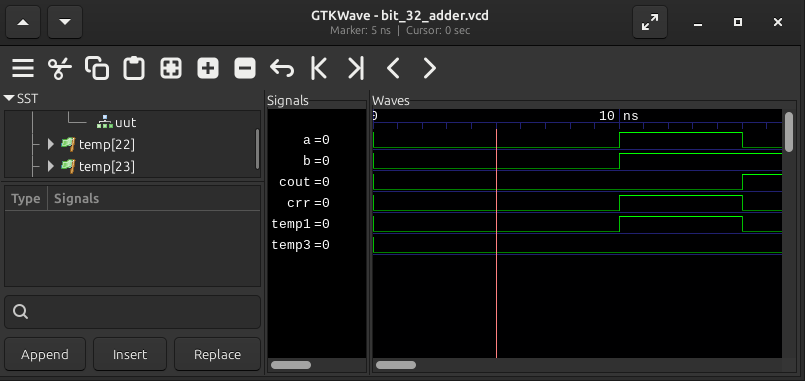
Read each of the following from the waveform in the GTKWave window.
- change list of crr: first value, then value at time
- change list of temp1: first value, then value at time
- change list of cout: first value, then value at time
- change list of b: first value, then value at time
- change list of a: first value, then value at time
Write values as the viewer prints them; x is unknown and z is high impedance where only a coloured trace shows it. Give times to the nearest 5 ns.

0, 1 at 10 ns, 0 at 15 ns
0, 1 at 10 ns, 0 at 15 ns
0, 1 at 15 ns
0, 1 at 10 ns
0, 1 at 10 ns, 0 at 15 ns
